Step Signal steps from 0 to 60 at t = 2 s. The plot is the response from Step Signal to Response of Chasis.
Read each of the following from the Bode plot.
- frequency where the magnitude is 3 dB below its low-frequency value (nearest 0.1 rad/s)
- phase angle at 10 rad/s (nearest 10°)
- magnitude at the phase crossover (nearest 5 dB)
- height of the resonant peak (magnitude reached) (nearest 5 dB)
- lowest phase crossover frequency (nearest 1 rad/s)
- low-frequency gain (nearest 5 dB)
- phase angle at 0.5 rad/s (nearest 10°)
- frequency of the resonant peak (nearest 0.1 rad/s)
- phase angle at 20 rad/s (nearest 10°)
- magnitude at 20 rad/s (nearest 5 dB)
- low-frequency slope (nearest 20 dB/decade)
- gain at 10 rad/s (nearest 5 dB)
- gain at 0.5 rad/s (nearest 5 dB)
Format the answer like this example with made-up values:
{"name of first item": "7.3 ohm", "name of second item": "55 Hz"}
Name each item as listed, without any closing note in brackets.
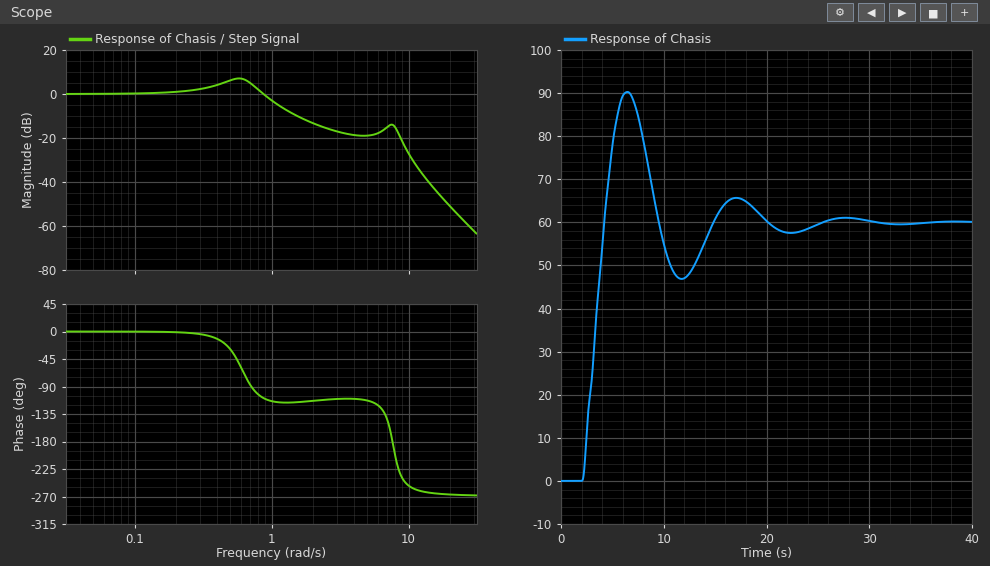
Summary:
{"frequency where the magnitude is 3 dB below its low-frequency value": "1.0 rad/s", "phase angle at 10 rad/s": "-250°", "magnitude at the phase crossover": "-15 dB", "height of the resonant peak (magnitude reached)": "5 dB", "lowest phase crossover frequency": "8 rad/s", "low-frequency gain": "0 dB", "phase angle at 0.5 rad/s": "-30°", "frequency of the resonant peak": "0.6 rad/s", "phase angle at 20 rad/s": "-270°", "magnitude at 20 rad/s": "-50 dB", "low-frequency slope": "0 dB/decade", "gain at 10 rad/s": "-25 dB", "gain at 0.5 rad/s": "5 dB"}
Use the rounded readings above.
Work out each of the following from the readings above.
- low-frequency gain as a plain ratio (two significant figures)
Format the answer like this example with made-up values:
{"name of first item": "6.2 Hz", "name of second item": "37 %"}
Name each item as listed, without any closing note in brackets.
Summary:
{"low-frequency gain as a plain ratio": "1.0"}
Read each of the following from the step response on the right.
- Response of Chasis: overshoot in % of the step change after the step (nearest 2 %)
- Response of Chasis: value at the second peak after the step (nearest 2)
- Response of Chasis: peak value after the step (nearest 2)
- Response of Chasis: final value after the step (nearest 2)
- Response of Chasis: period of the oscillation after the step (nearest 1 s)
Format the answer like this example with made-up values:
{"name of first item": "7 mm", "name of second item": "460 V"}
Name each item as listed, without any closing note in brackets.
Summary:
{"Response of Chasis: overshoot in % of the step change after the step": "50 %", "Response of Chasis: value at the second peak after the step": "66", "Response of Chasis: peak value after the step": "90", "Response of Chasis: final value after the step": "60", "Response of Chasis: period of the oscillation after the step": "11 s"}
